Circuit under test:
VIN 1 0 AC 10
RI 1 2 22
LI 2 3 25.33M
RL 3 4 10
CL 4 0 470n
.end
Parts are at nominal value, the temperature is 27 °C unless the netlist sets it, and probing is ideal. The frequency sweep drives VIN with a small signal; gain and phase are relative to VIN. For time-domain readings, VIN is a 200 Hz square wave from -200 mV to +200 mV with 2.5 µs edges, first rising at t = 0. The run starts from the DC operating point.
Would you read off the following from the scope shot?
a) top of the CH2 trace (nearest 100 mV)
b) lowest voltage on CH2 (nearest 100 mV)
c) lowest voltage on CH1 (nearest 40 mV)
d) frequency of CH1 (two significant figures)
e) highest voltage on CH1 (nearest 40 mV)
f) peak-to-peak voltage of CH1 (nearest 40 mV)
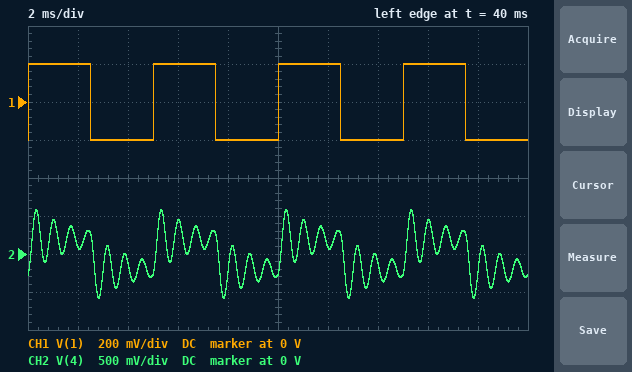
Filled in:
600 mV
-600 mV
-200 mV
200 Hz
200 mV
400 mV
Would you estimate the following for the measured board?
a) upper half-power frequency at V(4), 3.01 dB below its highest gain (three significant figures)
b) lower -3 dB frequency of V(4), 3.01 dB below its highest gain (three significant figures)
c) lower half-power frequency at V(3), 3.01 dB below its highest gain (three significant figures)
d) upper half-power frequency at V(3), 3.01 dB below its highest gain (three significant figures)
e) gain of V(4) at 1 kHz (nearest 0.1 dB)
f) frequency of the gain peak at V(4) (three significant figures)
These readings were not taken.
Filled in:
1.55 kHz
1.35 kHz
1.35 kHz
1.55 kHz
5.4 dB
1.45 kHz
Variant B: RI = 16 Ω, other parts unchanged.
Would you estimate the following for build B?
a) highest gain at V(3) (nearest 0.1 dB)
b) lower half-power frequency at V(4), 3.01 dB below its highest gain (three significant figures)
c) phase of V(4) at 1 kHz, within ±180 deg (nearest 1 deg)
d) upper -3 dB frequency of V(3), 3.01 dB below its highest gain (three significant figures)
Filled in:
19.0 dB
1.37 kHz
-8 deg
1.53 kHz
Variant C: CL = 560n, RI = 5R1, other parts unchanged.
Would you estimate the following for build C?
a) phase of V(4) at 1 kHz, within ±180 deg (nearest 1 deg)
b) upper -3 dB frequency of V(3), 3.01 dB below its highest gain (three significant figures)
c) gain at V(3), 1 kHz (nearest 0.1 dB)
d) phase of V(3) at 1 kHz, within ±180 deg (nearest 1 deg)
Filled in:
-7 deg
1.38 kHz
7.1 dB
-5 deg
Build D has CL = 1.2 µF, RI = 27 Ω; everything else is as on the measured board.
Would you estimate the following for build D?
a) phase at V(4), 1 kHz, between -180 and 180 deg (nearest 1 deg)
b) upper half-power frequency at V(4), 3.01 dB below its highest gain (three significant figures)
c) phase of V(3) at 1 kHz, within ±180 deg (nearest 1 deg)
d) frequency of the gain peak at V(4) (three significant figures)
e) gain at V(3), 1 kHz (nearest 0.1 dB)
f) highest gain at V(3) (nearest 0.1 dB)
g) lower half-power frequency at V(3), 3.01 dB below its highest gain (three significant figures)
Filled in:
-126 deg
1.01 kHz
-121 deg
898 Hz
9.3 dB
12.0 dB
772 Hz
